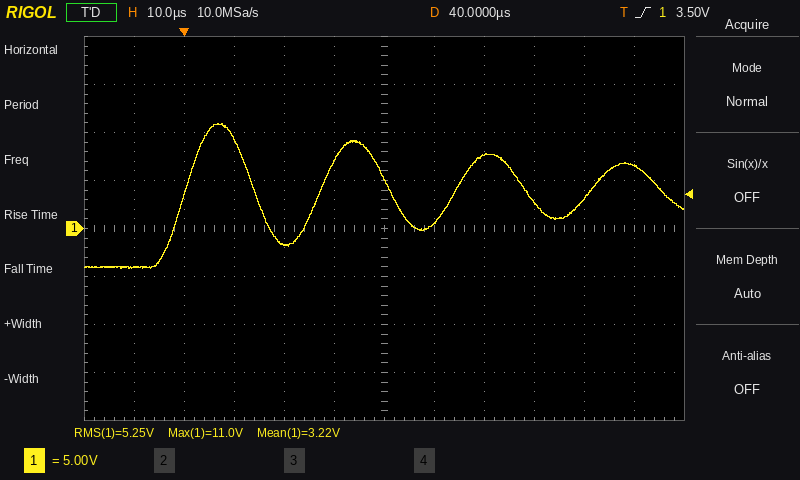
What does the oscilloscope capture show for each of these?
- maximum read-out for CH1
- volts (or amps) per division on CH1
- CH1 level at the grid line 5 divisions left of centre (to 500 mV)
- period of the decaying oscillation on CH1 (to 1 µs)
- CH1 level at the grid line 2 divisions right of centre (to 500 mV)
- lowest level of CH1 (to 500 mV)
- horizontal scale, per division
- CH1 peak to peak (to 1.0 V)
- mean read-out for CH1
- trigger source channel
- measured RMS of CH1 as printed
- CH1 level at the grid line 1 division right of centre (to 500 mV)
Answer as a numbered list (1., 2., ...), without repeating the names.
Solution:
1. 11.0 V
2. 5 V
3. -4.0 V
4. 27 µs
5. 7.5 V
6. -4.0 V
7. 10 µs
8. 15.0 V
9. 3.22 V
10. CH1
11. 5.25 V
12. 500 mV
